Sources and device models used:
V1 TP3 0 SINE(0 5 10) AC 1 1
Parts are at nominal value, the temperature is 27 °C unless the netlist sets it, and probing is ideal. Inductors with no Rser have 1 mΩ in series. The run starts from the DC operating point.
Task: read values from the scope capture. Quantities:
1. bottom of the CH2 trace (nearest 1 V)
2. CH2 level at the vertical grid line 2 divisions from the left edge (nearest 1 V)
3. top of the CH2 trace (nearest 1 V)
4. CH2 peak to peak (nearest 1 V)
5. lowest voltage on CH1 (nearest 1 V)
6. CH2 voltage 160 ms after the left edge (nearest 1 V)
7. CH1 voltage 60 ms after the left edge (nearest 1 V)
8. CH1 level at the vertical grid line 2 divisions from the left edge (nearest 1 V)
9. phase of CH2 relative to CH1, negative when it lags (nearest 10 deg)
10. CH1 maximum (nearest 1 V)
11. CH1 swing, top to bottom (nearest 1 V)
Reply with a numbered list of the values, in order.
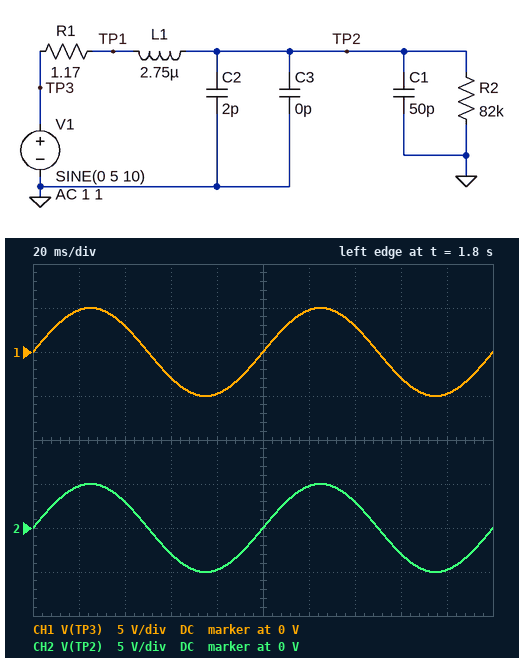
1. -5 V
2. 3 V
3. 5 V
4. 10 V
5. -5 V
6. -3 V
7. -3 V
8. 3 V
9. 0 deg
10. 5 V
11. 10 V
